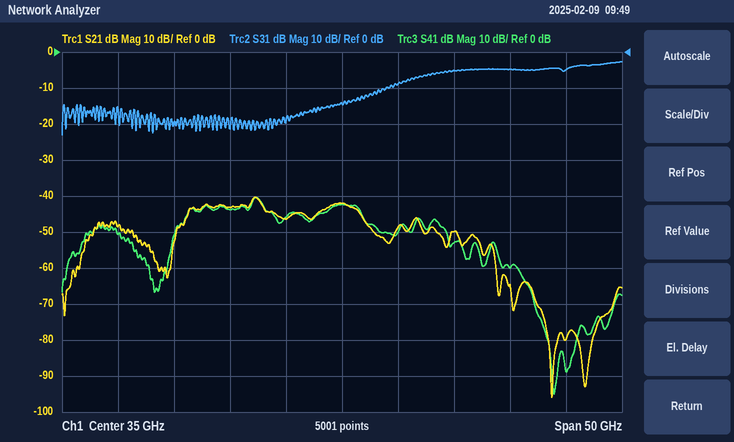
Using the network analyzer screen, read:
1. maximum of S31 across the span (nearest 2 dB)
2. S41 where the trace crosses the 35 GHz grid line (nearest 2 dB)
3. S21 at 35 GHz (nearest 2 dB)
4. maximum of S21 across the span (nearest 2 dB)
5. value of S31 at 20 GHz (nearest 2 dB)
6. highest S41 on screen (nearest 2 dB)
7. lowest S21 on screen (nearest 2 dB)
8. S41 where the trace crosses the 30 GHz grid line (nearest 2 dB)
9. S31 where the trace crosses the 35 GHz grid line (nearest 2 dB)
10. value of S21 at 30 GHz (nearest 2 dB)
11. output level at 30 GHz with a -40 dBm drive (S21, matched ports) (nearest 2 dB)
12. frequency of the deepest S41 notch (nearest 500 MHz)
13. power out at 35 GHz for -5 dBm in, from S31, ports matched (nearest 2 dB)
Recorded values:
-2 dB
-42 dB
-42 dB
-40 dB
-20 dB
-40 dB
-96 dB
-46 dB
-14 dB
-46 dB
-86 dBm
54.0 GHz
-20 dBm
